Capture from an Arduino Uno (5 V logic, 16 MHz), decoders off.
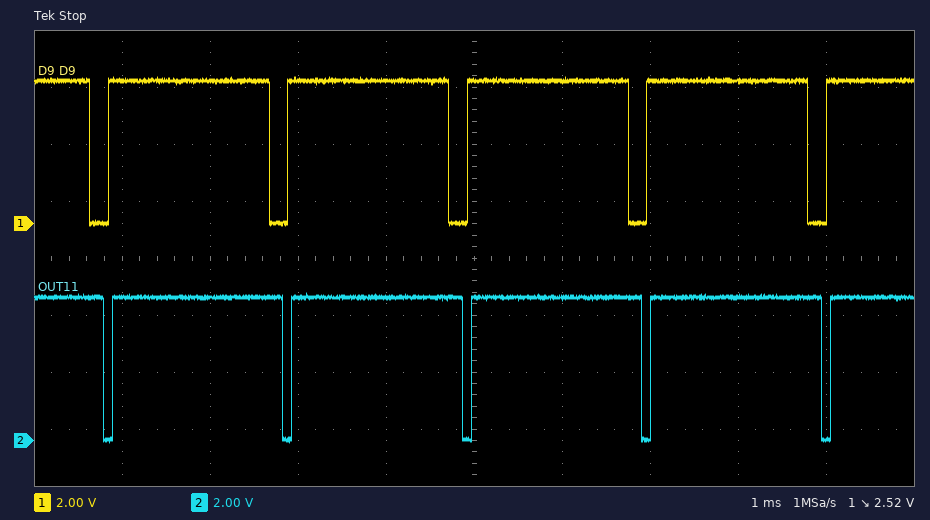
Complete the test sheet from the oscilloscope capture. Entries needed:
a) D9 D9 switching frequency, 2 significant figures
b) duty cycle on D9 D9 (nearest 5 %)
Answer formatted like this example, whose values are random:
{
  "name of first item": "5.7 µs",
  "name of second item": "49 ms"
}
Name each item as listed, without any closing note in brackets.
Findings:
{
  "D9 D9 switching frequency, 2 significant figures": "490 Hz",
  "duty cycle on D9 D9": "90 %"
}
